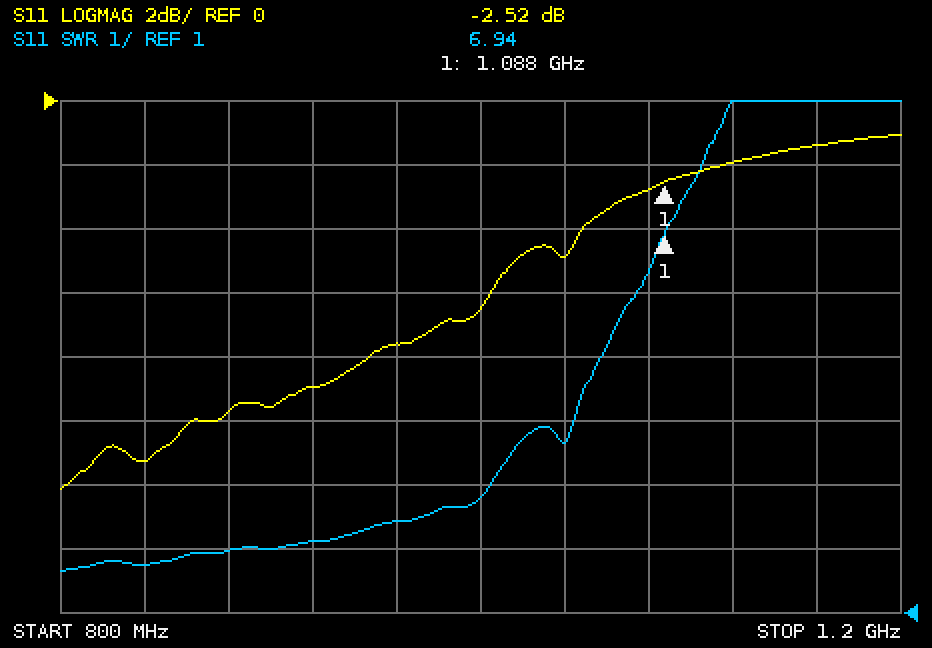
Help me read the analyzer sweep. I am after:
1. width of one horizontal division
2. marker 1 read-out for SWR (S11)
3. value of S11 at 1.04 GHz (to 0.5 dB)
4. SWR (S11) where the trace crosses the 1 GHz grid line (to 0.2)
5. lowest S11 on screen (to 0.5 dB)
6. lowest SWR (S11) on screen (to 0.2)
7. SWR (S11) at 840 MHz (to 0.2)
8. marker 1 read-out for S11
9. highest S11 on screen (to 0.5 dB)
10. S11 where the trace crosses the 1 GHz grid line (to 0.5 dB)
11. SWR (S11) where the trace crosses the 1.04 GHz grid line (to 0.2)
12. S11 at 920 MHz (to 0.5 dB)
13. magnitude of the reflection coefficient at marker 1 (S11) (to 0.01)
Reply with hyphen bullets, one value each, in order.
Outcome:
- 40 MHz
- 6.94
- -5.0 dB
- 2.8
- -12.0 dB
- 1.6
- 1.8
- -2.52 dB
- -1.0 dB
- -6.5 dB
- 3.6
- -9.0 dB
- 0.75
